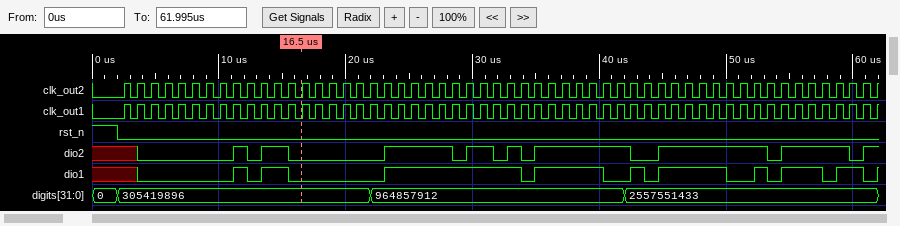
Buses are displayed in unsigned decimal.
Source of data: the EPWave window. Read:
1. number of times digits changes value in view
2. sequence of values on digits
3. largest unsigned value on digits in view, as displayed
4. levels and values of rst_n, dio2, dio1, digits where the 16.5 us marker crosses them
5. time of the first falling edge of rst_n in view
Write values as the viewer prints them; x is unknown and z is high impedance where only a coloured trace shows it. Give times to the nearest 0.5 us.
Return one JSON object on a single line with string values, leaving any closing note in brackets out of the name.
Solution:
{"number of times digits changes value in view": "3", "sequence of values on digits": "0, 305419896, 964857912, 2557551433", "largest unsigned value on digits in view, as displayed": "2557551433", "levels and values of rst_n, dio2, dio1, digits where the 16.5 us marker crosses them": "rst_n=0, dio2=0, dio1=0, digits=305419896", "time of the first falling edge of rst_n in view": "2 us"}
